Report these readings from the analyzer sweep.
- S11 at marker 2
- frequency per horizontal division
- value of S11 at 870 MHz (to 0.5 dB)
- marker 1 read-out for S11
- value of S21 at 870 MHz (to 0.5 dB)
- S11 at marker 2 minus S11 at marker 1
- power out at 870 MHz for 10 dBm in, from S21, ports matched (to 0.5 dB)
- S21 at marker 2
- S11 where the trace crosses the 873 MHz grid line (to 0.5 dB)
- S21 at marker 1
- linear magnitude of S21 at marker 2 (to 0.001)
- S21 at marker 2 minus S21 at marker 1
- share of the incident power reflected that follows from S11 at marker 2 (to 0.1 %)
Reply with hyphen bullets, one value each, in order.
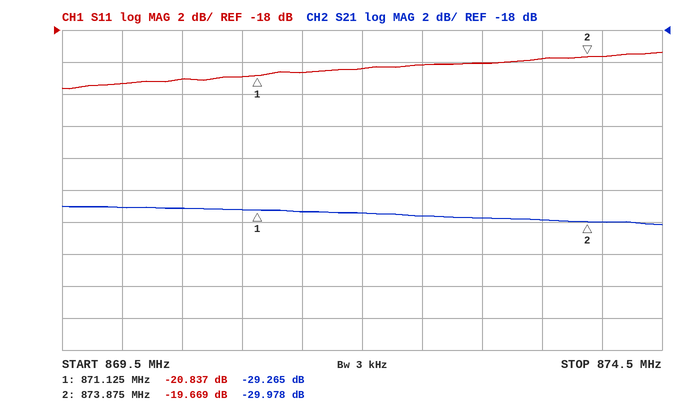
- -19.669 dB
- 500 kHz
- -21.5 dB
- -20.837 dB
- -29.0 dB
- 1.168 dB
- -19.0 dBm
- -29.978 dB
- -20.0 dB
- -29.265 dB
- 0.032
- -0.713 dB
- 1.1 %
